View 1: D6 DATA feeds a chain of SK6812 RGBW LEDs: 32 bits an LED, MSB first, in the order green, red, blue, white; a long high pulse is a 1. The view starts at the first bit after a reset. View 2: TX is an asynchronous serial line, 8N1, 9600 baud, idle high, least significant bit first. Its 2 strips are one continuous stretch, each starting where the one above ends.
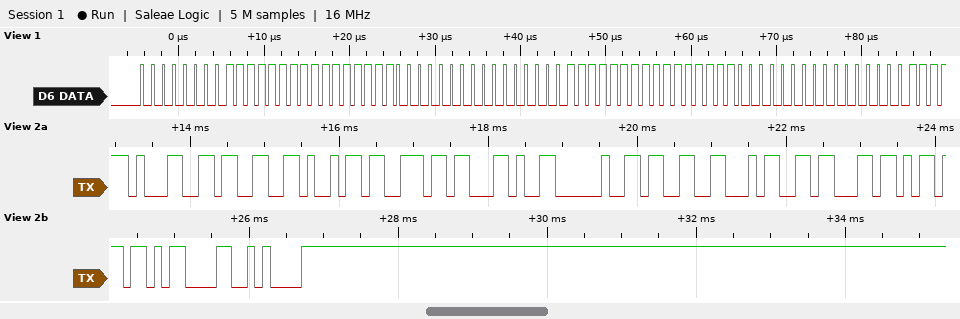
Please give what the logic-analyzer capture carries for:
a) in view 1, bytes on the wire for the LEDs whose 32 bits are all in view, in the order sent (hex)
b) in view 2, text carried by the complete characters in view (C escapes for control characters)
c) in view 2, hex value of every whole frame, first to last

00 FF FF 00 00 FF FF 00
"13in, 34cm\r\n"
31 33 69 6E 2C 20 33 34 63 6D 0D 0A
